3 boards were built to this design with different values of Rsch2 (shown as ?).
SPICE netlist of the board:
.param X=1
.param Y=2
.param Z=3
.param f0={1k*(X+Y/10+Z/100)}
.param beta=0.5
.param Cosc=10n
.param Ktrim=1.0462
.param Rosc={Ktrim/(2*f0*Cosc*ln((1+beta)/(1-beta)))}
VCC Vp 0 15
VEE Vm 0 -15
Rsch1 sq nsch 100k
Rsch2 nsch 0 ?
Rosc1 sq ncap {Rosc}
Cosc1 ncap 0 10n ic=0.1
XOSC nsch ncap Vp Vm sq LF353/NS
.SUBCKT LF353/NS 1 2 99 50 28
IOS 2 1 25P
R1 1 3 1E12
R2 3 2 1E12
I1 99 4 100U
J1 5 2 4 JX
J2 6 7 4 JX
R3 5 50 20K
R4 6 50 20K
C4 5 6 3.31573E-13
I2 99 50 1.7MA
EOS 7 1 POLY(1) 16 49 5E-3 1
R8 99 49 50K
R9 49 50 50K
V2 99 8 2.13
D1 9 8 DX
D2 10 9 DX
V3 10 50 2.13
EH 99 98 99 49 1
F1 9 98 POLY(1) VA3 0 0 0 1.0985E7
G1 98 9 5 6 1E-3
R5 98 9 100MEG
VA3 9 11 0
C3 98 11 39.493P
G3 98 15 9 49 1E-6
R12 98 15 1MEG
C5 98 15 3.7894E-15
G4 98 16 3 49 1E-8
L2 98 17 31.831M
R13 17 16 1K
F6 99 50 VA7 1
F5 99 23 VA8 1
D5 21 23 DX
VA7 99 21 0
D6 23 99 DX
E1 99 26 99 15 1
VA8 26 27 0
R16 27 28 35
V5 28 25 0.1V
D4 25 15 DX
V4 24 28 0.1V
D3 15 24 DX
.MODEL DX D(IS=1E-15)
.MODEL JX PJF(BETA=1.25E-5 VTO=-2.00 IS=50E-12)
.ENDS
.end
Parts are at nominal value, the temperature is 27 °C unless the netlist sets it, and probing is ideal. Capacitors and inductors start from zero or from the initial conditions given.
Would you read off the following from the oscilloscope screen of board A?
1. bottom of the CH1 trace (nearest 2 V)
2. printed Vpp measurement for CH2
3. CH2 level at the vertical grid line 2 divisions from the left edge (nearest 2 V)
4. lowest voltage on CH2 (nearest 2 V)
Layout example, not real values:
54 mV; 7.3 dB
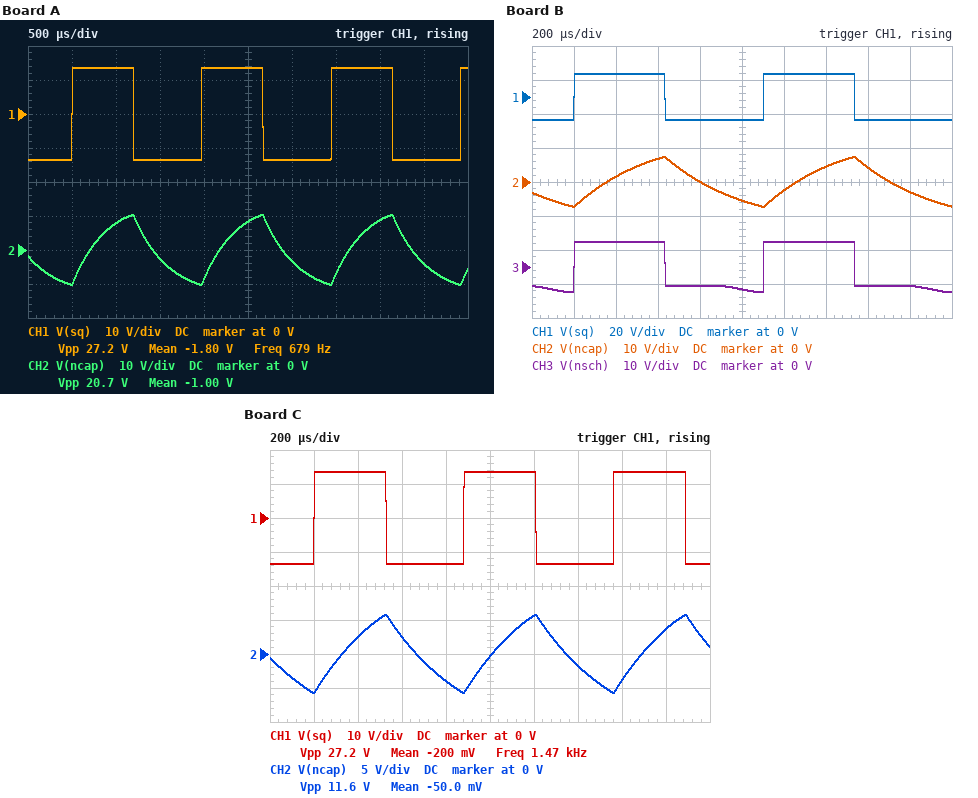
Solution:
-14 V; 20.7 V; 8 V; -10 V
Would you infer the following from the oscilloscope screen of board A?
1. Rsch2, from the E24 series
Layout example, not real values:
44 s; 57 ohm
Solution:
330 kΩ
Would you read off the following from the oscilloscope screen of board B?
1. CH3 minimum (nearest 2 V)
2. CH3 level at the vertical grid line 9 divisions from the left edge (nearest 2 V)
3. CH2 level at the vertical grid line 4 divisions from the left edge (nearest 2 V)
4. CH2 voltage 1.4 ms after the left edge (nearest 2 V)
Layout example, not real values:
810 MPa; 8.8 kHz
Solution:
-8 V; -6 V; 0 V; 4 V
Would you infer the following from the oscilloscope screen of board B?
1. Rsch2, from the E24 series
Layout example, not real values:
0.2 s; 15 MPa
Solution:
120 kΩ
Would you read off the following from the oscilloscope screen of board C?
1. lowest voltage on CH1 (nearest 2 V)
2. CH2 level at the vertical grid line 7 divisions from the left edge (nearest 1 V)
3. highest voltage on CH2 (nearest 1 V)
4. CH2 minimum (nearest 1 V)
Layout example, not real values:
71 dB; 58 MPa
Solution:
-14 V; -2 V; 6 V; -6 V
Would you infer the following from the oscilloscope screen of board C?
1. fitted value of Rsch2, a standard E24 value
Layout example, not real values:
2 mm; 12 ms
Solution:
75 kΩ
